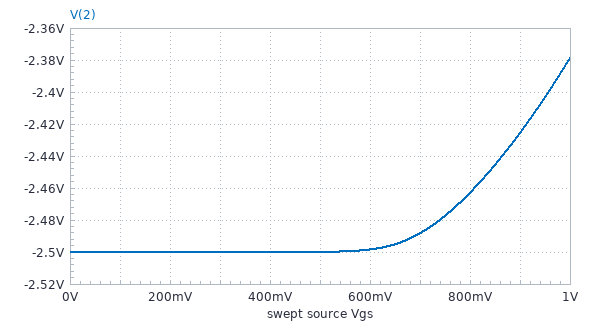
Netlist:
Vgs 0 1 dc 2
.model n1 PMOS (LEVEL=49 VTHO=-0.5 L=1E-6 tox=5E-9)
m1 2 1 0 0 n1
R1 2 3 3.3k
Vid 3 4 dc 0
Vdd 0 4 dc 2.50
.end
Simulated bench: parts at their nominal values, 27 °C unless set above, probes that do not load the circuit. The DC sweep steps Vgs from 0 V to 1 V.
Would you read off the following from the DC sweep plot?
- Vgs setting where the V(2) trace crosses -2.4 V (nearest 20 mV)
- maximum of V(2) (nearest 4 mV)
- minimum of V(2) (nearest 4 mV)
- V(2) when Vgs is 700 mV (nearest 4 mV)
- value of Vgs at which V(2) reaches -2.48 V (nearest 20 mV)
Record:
960 mV
-2.380 V
-2.500 V
-2.488 V
740 mV
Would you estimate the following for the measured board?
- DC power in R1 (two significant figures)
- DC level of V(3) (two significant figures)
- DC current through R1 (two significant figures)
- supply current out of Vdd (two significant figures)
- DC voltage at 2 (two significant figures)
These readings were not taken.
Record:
260 µW
-2.5 V
280 µA
280 µA
-1.6 V
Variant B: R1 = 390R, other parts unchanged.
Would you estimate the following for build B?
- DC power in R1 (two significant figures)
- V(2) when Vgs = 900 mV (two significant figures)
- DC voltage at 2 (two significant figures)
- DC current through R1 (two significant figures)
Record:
32 µW
-2.5 V
-2.4 V
290 µA
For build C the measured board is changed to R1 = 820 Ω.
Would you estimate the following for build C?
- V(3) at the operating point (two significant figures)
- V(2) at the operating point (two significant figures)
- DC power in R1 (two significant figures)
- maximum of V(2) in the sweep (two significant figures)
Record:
-2.5 V
-2.3 V
67 µW
-2.5 V
